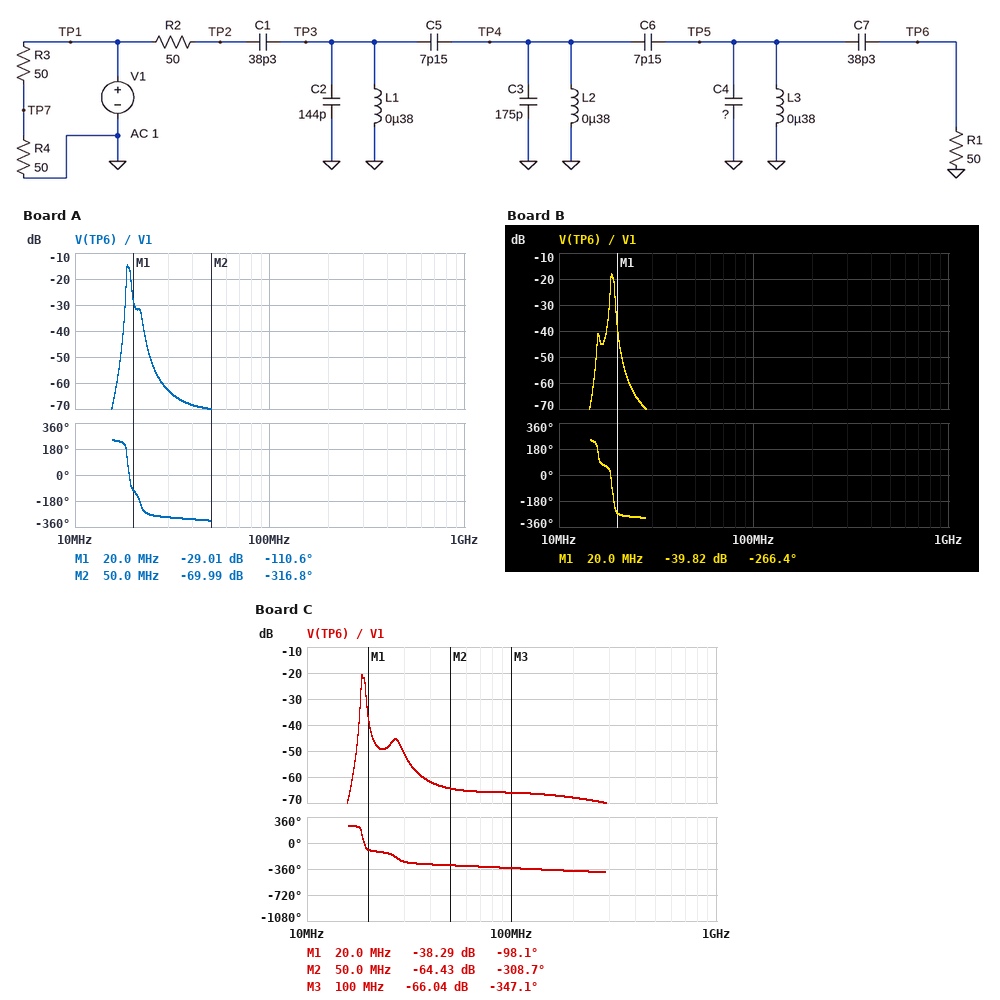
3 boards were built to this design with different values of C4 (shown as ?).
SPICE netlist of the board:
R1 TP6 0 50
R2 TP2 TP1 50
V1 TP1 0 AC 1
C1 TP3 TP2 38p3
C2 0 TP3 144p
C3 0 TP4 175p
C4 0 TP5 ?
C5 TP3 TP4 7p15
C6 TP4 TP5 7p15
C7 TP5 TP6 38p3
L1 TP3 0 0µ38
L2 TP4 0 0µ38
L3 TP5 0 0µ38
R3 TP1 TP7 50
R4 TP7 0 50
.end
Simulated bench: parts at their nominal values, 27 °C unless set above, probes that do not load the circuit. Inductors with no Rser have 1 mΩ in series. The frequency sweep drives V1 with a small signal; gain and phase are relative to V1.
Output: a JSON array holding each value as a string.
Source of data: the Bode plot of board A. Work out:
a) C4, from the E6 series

["100 pF"]
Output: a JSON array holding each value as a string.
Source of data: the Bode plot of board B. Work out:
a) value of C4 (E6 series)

["220 pF"]
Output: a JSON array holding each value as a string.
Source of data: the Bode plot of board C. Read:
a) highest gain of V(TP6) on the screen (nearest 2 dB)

["-20 dB"]
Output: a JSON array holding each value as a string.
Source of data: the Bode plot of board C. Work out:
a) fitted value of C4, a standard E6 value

["47 pF"]
